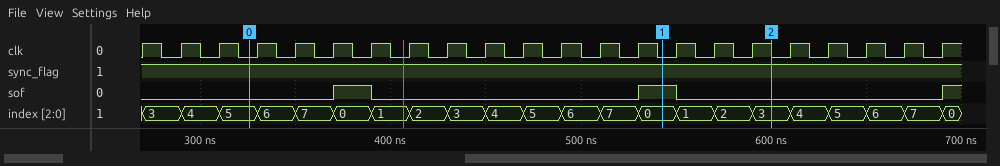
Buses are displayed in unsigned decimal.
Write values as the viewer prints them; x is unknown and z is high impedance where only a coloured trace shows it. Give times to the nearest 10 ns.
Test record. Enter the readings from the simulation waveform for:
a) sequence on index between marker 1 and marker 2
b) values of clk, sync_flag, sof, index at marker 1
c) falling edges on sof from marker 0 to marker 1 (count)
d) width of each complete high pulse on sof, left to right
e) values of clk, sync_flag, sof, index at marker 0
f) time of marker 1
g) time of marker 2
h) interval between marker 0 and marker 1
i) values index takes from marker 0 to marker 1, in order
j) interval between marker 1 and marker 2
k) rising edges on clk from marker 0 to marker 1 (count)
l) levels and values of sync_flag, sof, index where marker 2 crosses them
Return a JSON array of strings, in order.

["0, 1, 2, 3", "clk=0, sync_flag=1, sof=1, index=0", "1", "20 ns, 20 ns", "clk=0, sync_flag=1, sof=0, index=5", "540 ns", "600 ns", "220 ns", "5, 6, 7, 0, 1, 2, 3, 4, 5, 6, 7, 0", "60 ns", "11", "sync_flag=1, sof=0, index=3"]
